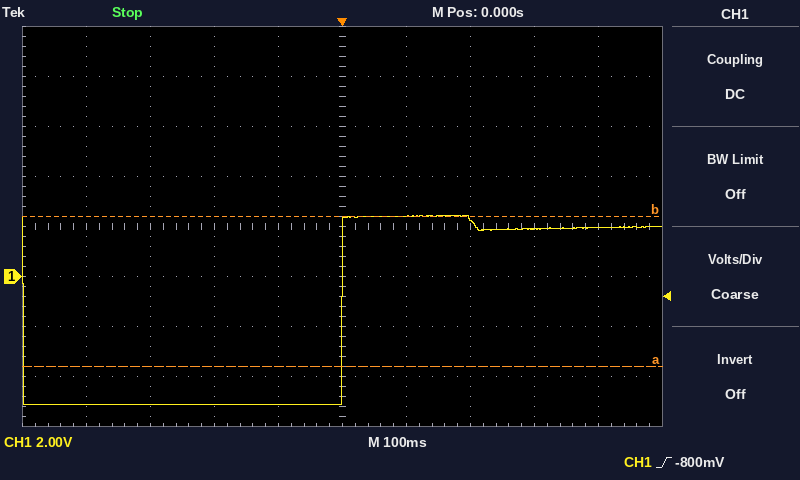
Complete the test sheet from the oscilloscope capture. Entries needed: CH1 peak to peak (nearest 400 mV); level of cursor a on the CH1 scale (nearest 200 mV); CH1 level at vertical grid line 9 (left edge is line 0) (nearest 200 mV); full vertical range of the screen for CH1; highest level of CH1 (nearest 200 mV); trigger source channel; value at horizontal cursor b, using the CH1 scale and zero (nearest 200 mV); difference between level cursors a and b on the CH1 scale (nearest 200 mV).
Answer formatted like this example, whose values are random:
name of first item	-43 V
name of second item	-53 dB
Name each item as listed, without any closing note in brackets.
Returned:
CH1 peak to peak	7.6 V
level of cursor a on the CH1 scale	-3.6 V
CH1 level at vertical grid line 9 (left edge is line 0)	2.0 V
full vertical range of the screen for CH1	16 V
highest level of CH1	2.4 V
trigger source channel	CH1
value at horizontal cursor b, using the CH1 scale and zero	2.4 V
difference between level cursors a and b on the CH1 scale	6.0 V
